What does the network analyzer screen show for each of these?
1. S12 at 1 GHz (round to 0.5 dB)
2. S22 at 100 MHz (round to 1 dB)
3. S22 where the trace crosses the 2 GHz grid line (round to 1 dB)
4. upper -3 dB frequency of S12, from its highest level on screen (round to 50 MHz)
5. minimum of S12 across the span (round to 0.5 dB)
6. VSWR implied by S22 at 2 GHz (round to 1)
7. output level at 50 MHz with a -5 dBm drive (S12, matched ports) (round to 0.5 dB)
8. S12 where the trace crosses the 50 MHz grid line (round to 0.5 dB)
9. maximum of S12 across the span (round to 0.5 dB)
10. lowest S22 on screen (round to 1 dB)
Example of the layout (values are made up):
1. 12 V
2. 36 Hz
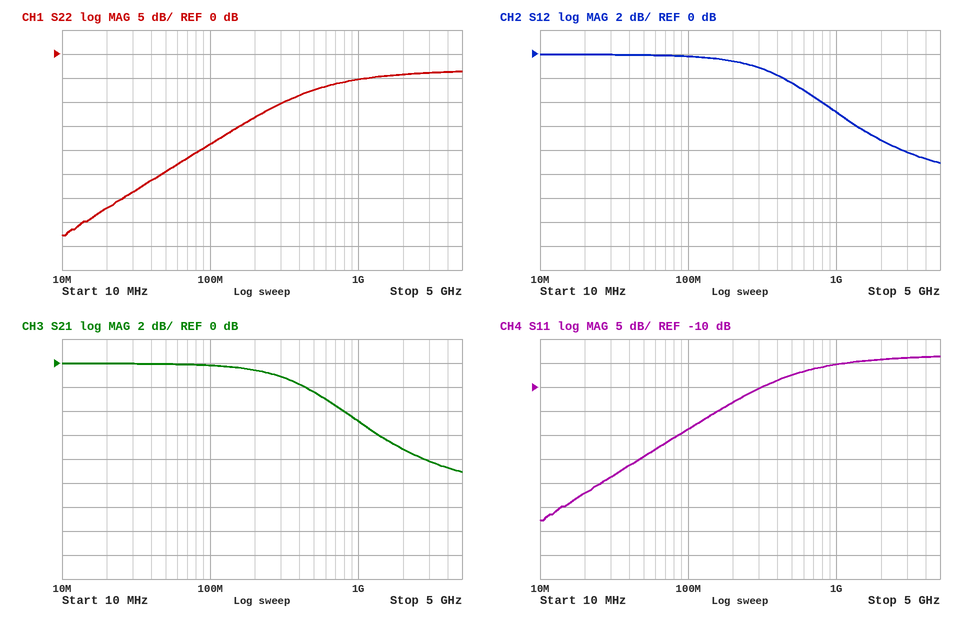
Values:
1. -5.0 dB
2. -19 dB
3. -4 dB
4. 600 MHz
5. -9.0 dB
6. 4
7. -5.0 dBm
8. 0.0 dB
9. 0.0 dB
10. -38 dB
